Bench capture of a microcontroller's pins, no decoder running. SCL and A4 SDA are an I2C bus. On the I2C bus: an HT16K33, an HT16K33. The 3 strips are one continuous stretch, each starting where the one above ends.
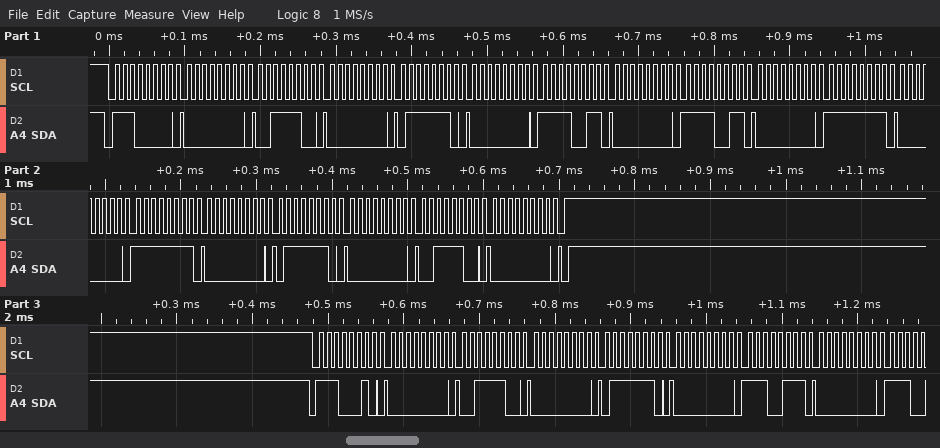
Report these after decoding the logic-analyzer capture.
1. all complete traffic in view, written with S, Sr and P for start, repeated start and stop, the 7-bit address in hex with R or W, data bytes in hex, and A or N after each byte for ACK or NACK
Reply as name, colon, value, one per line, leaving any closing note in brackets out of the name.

all complete traffic in view, written with S, Sr and P for start, repeated start and stop, the 7-bit address in hex with R or W, data bytes in hex, and A or N after each byte for ACK or NACK: S 70W A 00 A 3C A 00 A 7E A 00 A F3 A 00 A F3 A 00 A FF A 00 A FF A 00 A 7E A 00 A 3C A 00 A P S 71W A 00 A 3C A 00 A 7E A 00 A E7 A 00 A
